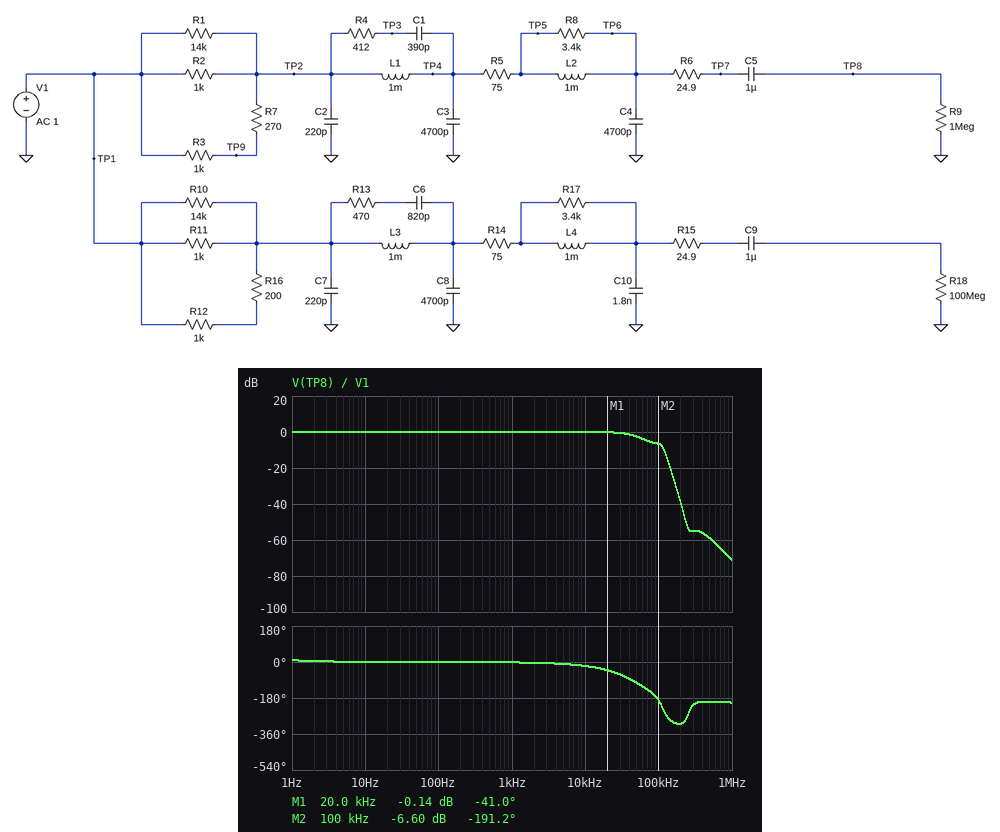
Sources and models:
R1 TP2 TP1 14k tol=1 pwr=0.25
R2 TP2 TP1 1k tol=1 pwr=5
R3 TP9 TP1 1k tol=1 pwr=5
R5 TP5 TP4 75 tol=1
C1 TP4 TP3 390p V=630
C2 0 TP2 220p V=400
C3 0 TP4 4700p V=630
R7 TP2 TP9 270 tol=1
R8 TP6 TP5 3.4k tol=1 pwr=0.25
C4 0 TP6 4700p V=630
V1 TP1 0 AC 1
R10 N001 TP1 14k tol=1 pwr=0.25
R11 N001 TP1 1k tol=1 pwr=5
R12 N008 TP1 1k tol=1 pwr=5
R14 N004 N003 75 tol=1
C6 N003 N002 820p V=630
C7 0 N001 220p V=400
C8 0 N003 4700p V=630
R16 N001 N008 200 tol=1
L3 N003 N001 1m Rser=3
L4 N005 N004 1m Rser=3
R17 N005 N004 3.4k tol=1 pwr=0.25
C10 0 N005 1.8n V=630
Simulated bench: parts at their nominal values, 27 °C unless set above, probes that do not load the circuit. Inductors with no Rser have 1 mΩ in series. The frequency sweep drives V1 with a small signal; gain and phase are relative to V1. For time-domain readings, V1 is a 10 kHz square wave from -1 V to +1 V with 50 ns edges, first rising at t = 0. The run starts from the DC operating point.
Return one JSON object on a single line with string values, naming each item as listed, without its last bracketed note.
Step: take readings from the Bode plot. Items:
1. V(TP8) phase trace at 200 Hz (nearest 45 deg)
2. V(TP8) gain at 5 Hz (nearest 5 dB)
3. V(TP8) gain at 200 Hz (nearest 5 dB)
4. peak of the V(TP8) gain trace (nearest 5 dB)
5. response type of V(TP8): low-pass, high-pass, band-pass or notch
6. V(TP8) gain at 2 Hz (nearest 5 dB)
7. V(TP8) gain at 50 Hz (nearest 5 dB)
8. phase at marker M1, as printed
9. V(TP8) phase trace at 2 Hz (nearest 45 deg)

{"V(TP8) phase trace at 200 Hz": "0 deg", "V(TP8) gain at 5 Hz": "0 dB", "V(TP8) gain at 200 Hz": "0 dB", "peak of the V(TP8) gain trace": "0 dB", "response type of V(TP8): low-pass, high-pass, band-pass or notch": "low-pass", "V(TP8) gain at 2 Hz": "0 dB", "V(TP8) gain at 50 Hz": "0 dB", "phase at marker M1, as printed": "-41.0 deg", "V(TP8) phase trace at 2 Hz": "0 deg"}
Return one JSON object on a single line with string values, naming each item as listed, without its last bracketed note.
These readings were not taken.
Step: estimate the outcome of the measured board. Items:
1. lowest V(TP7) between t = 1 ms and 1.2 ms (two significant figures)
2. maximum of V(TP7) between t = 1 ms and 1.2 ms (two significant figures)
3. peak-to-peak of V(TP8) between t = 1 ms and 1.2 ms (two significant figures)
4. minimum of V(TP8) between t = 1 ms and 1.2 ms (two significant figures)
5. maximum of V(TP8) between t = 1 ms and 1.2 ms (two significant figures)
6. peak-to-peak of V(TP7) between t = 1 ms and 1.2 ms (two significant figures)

{"lowest V(TP7) between t = 1 ms and 1.2 ms": "-1.1 V", "maximum of V(TP7) between t = 1 ms and 1.2 ms": "1.1 V", "peak-to-peak of V(TP8) between t = 1 ms and 1.2 ms": "2.2 V", "minimum of V(TP8) between t = 1 ms and 1.2 ms": "-85 mV", "maximum of V(TP8) between t = 1 ms and 1.2 ms": "2.1 V", "peak-to-peak of V(TP7) between t = 1 ms and 1.2 ms": "2.2 V"}
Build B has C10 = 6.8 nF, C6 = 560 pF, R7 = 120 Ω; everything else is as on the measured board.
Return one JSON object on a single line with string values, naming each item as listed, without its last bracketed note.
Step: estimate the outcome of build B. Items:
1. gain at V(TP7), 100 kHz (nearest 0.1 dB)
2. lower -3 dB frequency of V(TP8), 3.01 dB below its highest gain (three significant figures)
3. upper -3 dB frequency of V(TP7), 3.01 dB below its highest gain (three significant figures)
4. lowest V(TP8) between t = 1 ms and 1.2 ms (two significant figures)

{"gain at V(TP7), 100 kHz": "-6.4 dB", "lower -3 dB frequency of V(TP8), 3.01 dB below its highest gain": "161 mHz", "upper -3 dB frequency of V(TP7), 3.01 dB below its highest gain": "56.6 kHz", "lowest V(TP8) between t = 1 ms and 1.2 ms": "-110 mV"}
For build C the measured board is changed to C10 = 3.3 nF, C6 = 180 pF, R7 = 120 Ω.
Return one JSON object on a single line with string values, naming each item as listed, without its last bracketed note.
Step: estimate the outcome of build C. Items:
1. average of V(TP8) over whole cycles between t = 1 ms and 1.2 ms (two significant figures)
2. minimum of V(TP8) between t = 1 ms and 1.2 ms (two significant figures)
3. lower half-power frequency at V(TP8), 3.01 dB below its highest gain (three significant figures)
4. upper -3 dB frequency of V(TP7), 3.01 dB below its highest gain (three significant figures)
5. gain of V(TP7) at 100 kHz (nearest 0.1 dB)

{"average of V(TP8) over whole cycles between t = 1 ms and 1.2 ms": "1.0 V", "minimum of V(TP8) between t = 1 ms and 1.2 ms": "-110 mV", "lower half-power frequency at V(TP8), 3.01 dB below its highest gain": "161 mHz", "upper -3 dB frequency of V(TP7), 3.01 dB below its highest gain": "56.6 kHz", "gain of V(TP7) at 100 kHz": "-6.4 dB"}
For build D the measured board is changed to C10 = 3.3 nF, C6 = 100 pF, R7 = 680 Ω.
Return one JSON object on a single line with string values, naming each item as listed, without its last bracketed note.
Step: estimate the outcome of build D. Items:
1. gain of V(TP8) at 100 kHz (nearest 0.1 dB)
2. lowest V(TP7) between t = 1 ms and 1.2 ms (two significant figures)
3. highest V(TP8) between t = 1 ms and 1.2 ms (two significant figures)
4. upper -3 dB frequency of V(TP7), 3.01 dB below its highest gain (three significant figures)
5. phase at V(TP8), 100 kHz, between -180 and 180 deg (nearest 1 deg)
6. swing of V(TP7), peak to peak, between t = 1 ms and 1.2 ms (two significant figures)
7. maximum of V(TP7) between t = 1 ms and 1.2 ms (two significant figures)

{"gain of V(TP8) at 100 kHz": "-7.0 dB", "lowest V(TP7) between t = 1 ms and 1.2 ms": "-1.0 V", "highest V(TP8) between t = 1 ms and 1.2 ms": "2.0 V", "upper -3 dB frequency of V(TP7), 3.01 dB below its highest gain": "46.7 kHz", "phase at V(TP8), 100 kHz, between -180 and 180 deg": "170 deg", "swing of V(TP7), peak to peak, between t = 1 ms and 1.2 ms": "2.1 V", "maximum of V(TP7) between t = 1 ms and 1.2 ms": "1.0 V"}
